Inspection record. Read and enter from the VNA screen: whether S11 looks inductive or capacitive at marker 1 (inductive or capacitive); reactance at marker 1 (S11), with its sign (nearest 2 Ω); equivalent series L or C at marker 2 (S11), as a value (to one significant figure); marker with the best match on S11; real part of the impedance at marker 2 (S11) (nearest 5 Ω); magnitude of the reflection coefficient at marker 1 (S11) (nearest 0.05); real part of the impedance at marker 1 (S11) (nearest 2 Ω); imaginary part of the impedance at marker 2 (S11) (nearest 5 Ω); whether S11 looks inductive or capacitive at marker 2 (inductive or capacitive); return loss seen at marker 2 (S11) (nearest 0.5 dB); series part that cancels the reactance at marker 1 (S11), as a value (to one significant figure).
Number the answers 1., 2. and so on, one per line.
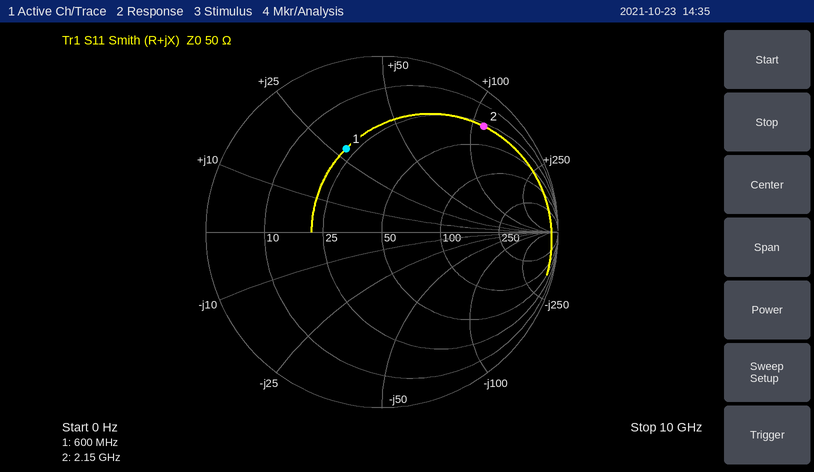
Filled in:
1. inductive
2. +28 Ω
3. 8 nH
4. marker 1
5. 30 Ω
6. 0.50
7. 22 Ω
8. +110 Ω
9. inductive
10. 1.5 dB
11. 9 pF
